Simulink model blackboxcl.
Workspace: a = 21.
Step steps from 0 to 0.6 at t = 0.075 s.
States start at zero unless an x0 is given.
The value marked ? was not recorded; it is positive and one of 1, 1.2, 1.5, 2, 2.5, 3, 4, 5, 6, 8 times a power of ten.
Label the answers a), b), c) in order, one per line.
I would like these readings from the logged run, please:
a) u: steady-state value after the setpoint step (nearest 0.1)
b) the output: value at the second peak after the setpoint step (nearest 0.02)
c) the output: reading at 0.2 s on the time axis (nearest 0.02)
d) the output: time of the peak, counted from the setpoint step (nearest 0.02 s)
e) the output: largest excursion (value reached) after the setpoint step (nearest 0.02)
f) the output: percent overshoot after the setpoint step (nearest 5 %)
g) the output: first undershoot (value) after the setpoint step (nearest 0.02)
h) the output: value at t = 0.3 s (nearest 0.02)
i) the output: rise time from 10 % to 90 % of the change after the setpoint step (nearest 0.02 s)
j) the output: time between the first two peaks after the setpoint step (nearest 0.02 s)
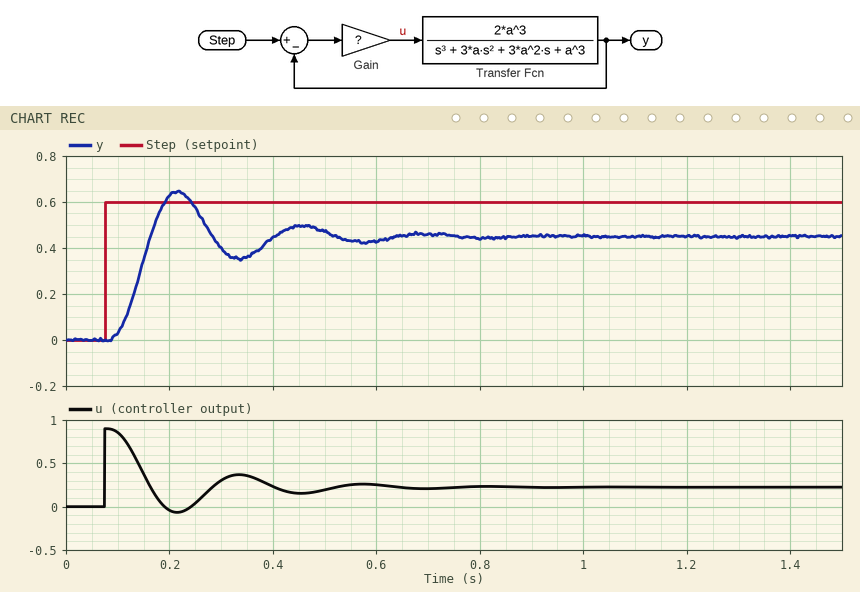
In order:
a) 0.2
b) 0.50
c) 0.62
d) 0.14 s
e) 0.64
f) 45 %
g) 0.36
h) 0.40
i) 0.06 s
j) 0.24 s
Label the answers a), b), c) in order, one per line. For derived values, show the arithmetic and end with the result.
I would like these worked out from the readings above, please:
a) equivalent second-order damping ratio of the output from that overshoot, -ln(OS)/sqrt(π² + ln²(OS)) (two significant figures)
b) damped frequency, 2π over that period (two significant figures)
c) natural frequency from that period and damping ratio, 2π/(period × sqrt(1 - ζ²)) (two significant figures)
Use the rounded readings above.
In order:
a) ln(0.45) = -0.799; 0.799 / sqrt(9.870 + 0.638) = 0.25
b) 2π / 0.24 = 26 rad/s
c) 2π / (0.24 × sqrt(1 - 0.25²)) = 27 rad/s
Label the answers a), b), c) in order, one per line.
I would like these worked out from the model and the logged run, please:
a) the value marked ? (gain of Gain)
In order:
a) 1.5
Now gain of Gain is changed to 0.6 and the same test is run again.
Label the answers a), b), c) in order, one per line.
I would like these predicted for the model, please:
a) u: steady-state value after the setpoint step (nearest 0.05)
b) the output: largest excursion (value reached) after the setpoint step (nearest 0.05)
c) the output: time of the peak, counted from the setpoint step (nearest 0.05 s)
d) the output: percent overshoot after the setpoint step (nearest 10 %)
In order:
a) 0.15
b) 0.40
c) 0.20 s
d) 20 %
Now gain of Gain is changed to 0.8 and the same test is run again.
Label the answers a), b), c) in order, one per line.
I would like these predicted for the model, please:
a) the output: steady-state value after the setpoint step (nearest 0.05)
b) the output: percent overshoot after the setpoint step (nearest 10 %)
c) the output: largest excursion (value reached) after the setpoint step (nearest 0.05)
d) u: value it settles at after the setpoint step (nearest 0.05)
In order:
a) 0.35
b) 20 %
c) 0.45
d) 0.20
